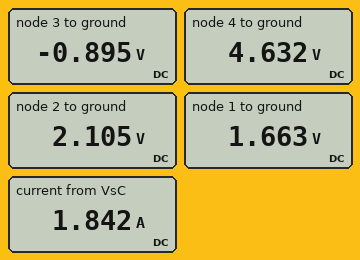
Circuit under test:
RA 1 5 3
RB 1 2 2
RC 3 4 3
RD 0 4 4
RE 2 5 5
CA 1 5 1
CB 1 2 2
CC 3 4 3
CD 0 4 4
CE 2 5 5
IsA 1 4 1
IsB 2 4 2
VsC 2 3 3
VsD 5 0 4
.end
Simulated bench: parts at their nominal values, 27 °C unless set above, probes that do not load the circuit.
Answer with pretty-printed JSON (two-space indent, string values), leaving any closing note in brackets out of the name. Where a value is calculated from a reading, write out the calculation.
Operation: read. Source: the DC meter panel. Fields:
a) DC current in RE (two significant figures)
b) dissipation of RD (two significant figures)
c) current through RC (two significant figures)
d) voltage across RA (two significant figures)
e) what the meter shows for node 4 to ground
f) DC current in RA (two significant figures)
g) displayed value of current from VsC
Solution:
{
  "DC current in RE": "(4 V - 2.105 V) / 5 Ω = 380 mA",
  "dissipation of RD": "(4.632 V)^2 / 4 Ω = 5.4 W",
  "current through RC": "(4.632 V - (-895 mV)) / 3 Ω = 1.8 A",
  "voltage across RA": "4 V - 1.663 V = 2.3 V",
  "what the meter shows for node 4 to ground": "4.632 V",
  "DC current in RA": "(4 V - 1.663 V) / 3 Ω = 780 mA",
  "displayed value of current from VsC": "1.842 A"
}
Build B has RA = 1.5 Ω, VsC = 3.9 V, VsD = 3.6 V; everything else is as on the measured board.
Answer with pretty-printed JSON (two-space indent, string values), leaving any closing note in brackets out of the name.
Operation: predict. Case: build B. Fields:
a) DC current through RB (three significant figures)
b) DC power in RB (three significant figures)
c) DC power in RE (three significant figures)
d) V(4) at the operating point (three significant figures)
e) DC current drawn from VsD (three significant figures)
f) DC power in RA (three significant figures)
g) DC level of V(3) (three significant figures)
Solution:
{
  "DC current through RB": "123 mA",
  "DC power in RB": "30.4 mW",
  "DC power in RE": "228 mW",
  "V(4) at the operating point": "4.36 V",
  "DC current drawn from VsD": "1.09 A",
  "DC power in RA": "1.15 W",
  "DC level of V(3)": "-1.37 V"
}
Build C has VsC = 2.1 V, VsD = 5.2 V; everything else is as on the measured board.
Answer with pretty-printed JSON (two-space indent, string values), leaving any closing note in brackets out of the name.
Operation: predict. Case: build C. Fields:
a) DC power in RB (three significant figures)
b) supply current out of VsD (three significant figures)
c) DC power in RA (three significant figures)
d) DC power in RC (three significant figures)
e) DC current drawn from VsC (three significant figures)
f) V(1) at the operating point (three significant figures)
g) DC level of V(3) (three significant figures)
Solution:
{
  "DC power in RB": "24.4 mW",
  "supply current out of VsD": "1.38 A",
  "DC power in RA": "2.37 W",
  "DC power in RC": "7.88 W",
  "DC current drawn from VsC": "1.62 A",
  "V(1) at the operating point": "2.53 V",
  "DC level of V(3)": "653 mV"
}
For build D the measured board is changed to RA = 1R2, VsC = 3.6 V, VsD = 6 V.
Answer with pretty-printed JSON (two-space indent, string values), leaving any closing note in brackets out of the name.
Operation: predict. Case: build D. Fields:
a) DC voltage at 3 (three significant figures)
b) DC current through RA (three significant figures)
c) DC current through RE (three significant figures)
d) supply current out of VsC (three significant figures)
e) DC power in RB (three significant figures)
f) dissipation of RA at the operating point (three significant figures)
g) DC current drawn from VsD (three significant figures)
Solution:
{
  "DC voltage at 3": "869 mV",
  "DC current through RA": "1.10 A",
  "DC current through RE": "306 mA",
  "supply current out of VsC": "1.59 A",
  "DC power in RB": "21.4 mW",
  "dissipation of RA at the operating point": "1.46 W",
  "DC current drawn from VsD": "1.41 A"
}
